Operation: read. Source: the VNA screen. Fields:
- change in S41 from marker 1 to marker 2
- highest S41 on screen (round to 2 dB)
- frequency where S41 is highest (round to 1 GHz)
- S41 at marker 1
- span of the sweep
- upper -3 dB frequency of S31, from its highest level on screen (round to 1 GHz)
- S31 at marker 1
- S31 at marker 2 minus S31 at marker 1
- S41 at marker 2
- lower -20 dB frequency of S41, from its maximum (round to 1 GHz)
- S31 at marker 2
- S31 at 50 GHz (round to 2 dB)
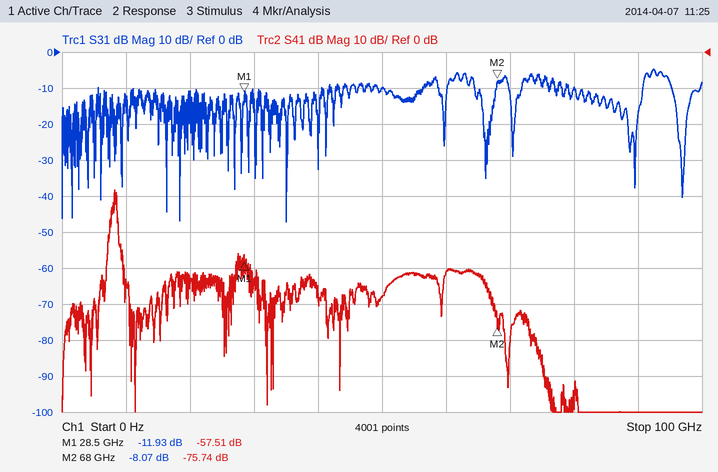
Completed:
-18.23 dB
-38 dB
8 GHz
-57.51 dB
100 GHz
95 GHz
-11.93 dB
3.86 dB
-75.74 dB
7 GHz
-8.07 dB
-10 dB
